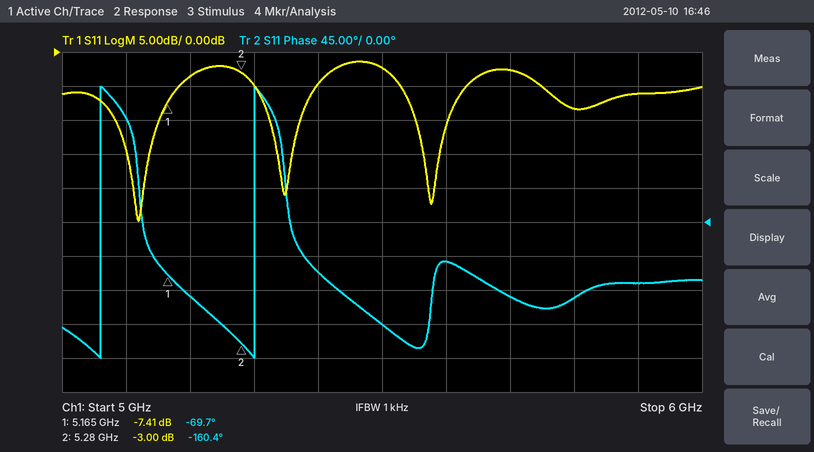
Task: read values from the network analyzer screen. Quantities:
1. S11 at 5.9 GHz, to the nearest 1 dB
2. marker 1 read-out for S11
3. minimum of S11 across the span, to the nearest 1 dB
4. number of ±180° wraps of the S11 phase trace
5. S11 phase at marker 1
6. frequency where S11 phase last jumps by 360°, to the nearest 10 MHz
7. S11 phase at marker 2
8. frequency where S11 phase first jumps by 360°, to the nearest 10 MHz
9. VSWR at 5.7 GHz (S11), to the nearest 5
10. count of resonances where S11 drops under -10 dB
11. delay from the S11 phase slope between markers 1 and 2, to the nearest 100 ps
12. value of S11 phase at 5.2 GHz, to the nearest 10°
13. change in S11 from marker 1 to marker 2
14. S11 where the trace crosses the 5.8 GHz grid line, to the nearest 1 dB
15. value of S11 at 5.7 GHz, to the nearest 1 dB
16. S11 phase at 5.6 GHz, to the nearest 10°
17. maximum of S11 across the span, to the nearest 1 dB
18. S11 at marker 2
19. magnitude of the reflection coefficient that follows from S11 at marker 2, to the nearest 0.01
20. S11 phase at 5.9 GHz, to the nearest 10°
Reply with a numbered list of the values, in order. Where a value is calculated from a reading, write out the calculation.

1. -6 dB
2. -7.41 dB
3. -25 dB
4. 2
5. -69.7°
6. 5.30 GHz
7. -160.4°
8. 5.06 GHz
9. |Γ| = 10^(-3/20) = 0.7079; VSWR = (1 + 0.7079)/(1 − 0.7079) ≈ 5.85, so 5 to the nearest 5
10. 3
11. −(-160.4° − (-69.7°))/(360° × 115 MHz) ≈ 2.2 ns
12. -100°
13. -3 − (-7.41) = 4.41 dB
14. -8 dB
15. -3 dB
16. -50°
17. -1 dB
18. -3.00 dB
19. 10^(-3/20) ≈ 0.71
20. -80°
